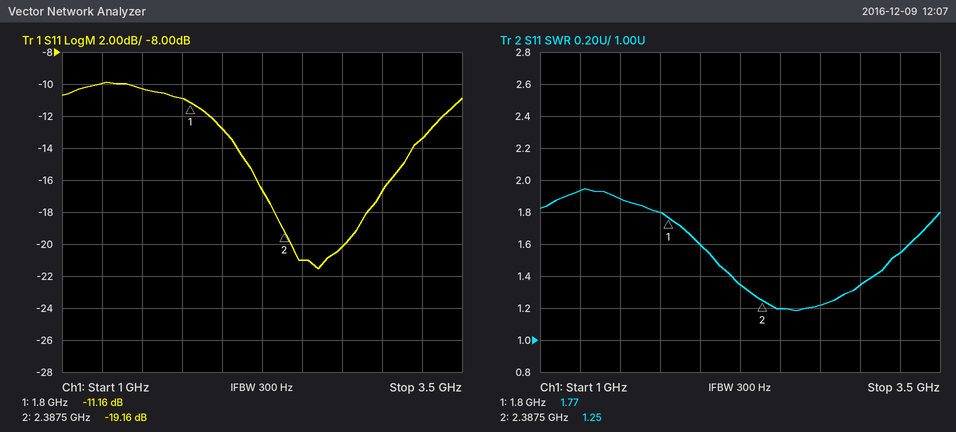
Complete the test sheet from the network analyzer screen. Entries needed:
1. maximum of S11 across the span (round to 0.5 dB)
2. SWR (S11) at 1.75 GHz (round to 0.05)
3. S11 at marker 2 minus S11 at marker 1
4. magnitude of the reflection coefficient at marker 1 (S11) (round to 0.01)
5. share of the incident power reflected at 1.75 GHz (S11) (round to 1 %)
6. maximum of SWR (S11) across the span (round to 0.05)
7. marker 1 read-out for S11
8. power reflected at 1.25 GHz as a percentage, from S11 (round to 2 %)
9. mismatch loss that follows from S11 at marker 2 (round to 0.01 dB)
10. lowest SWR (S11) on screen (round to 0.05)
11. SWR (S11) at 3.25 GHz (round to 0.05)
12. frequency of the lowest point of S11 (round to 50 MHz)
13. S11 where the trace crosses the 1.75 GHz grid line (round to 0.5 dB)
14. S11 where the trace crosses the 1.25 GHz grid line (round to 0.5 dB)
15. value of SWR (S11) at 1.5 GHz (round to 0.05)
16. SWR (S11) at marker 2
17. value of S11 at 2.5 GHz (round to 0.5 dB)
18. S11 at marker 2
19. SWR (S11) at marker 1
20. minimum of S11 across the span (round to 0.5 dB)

-10.0 dB
1.80
-8.00 dB
0.28
8 %
1.95
-11.16 dB
10 %
0.05 dB
1.20
1.55
2.60 GHz
-11.0 dB
-10.0 dB
1.90
1.25
-21.0 dB
-19.16 dB
1.77
-21.5 dB
